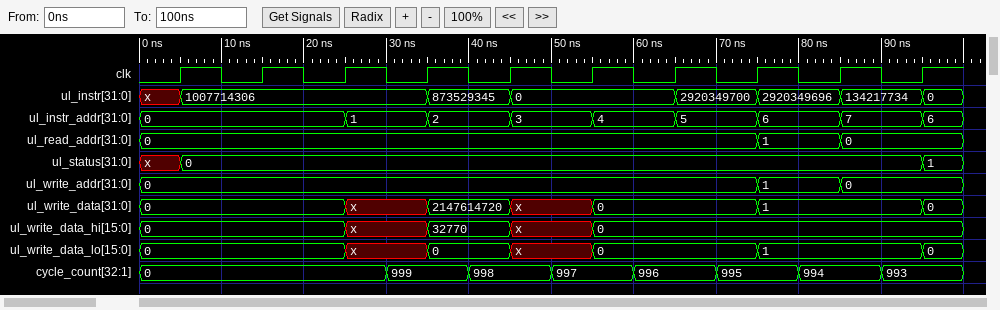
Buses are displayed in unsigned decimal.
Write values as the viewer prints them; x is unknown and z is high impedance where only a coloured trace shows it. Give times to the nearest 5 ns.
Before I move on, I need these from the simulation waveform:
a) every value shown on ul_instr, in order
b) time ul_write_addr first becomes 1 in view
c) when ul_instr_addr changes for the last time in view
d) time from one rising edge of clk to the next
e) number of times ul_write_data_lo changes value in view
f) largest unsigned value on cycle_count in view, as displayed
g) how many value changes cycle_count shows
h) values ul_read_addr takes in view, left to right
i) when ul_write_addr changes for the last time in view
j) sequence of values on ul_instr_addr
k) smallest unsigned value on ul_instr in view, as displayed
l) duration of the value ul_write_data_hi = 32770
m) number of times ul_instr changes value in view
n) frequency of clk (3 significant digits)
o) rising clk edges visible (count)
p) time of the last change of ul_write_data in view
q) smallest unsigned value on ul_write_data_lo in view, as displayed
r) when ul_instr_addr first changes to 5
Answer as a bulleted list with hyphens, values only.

- x, 1007714306, 873529345, 0, 2920349700, 2920349696, 134217734, 0
- 75 ns
- 95 ns
- 10 ns
- 6
- 999
- 7
- 0, 1, 0
- 85 ns
- 0, 1, 2, 3, 4, 5, 6, 7, 6
- 0
- 10 ns
- 7
- 100 MHz
- 10
- 95 ns
- 0
- 65 ns
